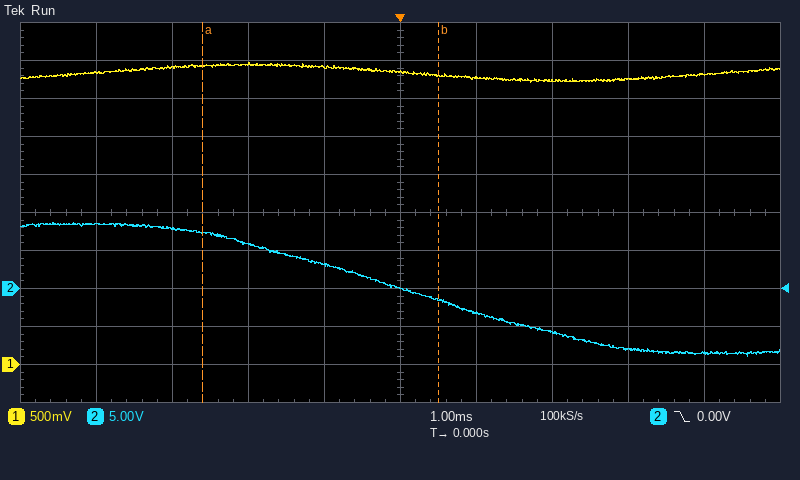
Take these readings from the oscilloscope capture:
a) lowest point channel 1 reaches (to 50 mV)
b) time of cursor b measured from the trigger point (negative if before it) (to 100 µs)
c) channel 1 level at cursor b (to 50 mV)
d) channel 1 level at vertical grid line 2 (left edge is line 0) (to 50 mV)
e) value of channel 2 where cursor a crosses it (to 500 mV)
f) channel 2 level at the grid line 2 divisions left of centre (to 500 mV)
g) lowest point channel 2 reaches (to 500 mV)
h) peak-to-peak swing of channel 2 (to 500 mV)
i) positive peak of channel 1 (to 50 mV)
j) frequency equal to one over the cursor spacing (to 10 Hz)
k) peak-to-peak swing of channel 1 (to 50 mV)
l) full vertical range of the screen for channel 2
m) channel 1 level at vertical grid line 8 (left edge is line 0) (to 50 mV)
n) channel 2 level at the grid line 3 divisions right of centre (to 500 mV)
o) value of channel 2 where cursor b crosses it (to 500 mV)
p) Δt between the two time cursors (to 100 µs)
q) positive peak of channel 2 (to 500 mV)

3.70 V
+500 µs
3.80 V
3.90 V
7.5 V
6.0 V
-9.0 V
17.5 V
3.95 V
320 Hz
250 mV
50 V
3.75 V
-8.0 V
-1.5 V
3.1 ms
8.5 V
